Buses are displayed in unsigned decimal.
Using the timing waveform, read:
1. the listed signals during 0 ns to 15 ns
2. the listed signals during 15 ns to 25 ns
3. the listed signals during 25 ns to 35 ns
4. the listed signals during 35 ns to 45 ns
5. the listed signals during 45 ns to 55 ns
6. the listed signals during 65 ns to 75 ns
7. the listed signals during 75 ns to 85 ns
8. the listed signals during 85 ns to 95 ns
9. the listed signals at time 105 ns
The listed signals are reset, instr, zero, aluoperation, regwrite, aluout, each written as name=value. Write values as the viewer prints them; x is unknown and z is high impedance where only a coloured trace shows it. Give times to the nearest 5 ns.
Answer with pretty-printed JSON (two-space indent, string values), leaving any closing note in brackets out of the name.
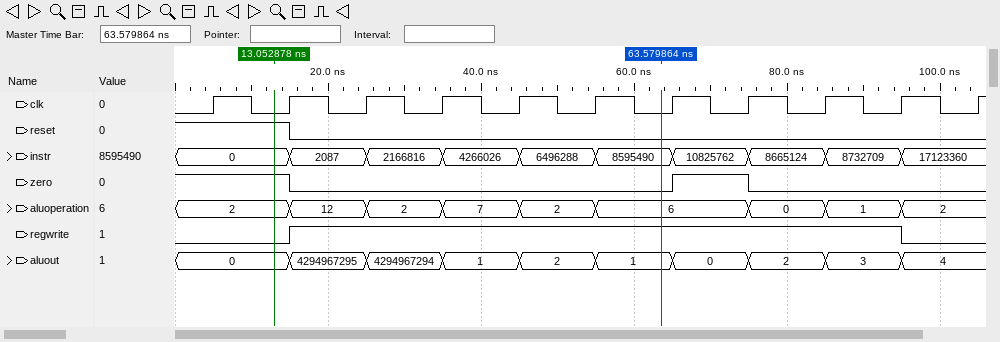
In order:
{
  "the listed signals during 0 ns to 15 ns": "reset=1, instr=0, zero=1, aluoperation=2, regwrite=0, aluout=0",
  "the listed signals during 15 ns to 25 ns": "reset=0, instr=2087, zero=0, aluoperation=12, regwrite=1, aluout=4294967295",
  "the listed signals during 25 ns to 35 ns": "reset=0, instr=2166816, zero=0, aluoperation=2, regwrite=1, aluout=4294967294",
  "the listed signals during 35 ns to 45 ns": "reset=0, instr=4266026, zero=0, aluoperation=7, regwrite=1, aluout=1",
  "the listed signals during 45 ns to 55 ns": "reset=0, instr=6496288, zero=0, aluoperation=2, regwrite=1, aluout=2",
  "the listed signals during 65 ns to 75 ns": "reset=0, instr=10825762, zero=1, aluoperation=6, regwrite=1, aluout=0",
  "the listed signals during 75 ns to 85 ns": "reset=0, instr=8665124, zero=0, aluoperation=0, regwrite=1, aluout=2",
  "the listed signals during 85 ns to 95 ns": "reset=0, instr=8732709, zero=0, aluoperation=1, regwrite=1, aluout=3",
  "the listed signals at time 105 ns": "reset=0, instr=17123360, zero=0, aluoperation=2, regwrite=0, aluout=4"
}
